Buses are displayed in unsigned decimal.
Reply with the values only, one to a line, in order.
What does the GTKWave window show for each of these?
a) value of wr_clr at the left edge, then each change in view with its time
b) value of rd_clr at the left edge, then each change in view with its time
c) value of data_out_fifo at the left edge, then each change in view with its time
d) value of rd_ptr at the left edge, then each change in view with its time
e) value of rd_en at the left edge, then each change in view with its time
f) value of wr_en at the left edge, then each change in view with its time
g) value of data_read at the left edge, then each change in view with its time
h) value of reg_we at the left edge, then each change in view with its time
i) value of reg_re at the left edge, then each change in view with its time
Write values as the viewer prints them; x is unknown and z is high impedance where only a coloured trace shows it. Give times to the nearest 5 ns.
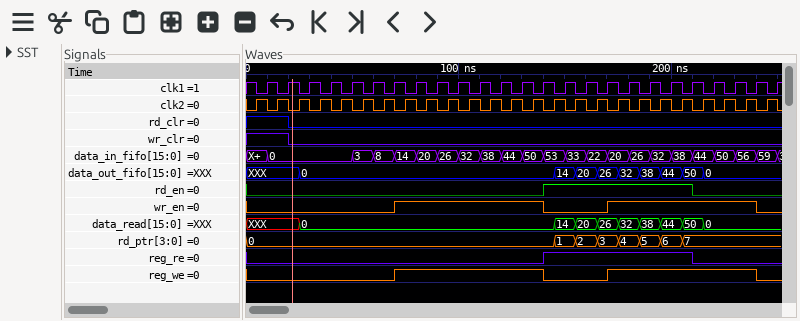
1, 0 at 20 ns
1, 0 at 20 ns
XXX, 0 at 25 ns, 14 at 145 ns, 20 at 155 ns, 26 at 165 ns, 32 at 175 ns, 38 at 185 ns, 44 at 195 ns, 50 at 205 ns, 0 at 215 ns
0, 1 at 145 ns, 2 at 155 ns, 3 at 165 ns, 4 at 175 ns, 5 at 185 ns, 6 at 195 ns, 7 at 205 ns
0, 1 at 140 ns, 0 at 210 ns
0, 1 at 70 ns, 0 at 140 ns, 1 at 170 ns, 0 at 240 ns
XXX, 0 at 25 ns, 14 at 145 ns, 20 at 155 ns, 26 at 165 ns, 32 at 175 ns, 38 at 185 ns, 44 at 195 ns, 50 at 205 ns, 0 at 215 ns
0, 1 at 70 ns, 0 at 140 ns, 1 at 170 ns, 0 at 240 ns
0, 1 at 140 ns, 0 at 210 ns
